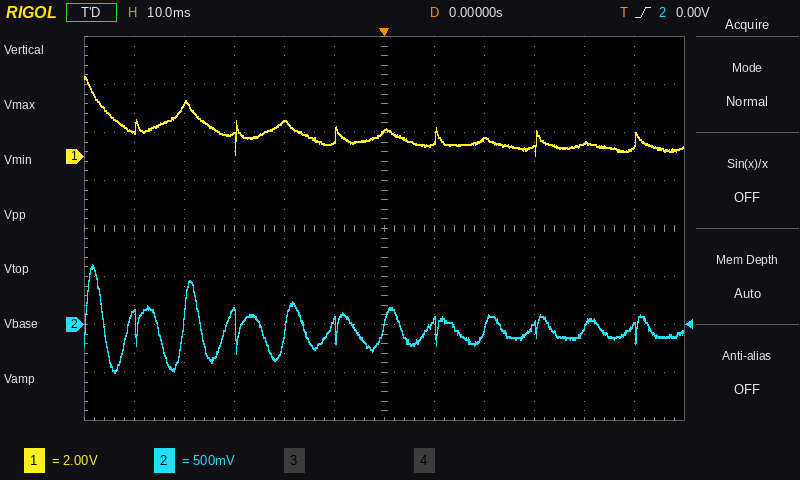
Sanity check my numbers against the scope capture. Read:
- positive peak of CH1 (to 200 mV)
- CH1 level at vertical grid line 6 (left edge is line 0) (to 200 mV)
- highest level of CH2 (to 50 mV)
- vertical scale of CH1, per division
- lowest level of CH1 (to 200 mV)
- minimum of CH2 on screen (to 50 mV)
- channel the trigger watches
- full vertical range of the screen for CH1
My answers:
3.4 V
1.0 V
600 mV
2 V
0.0 V
-500 mV
CH2
16 V
